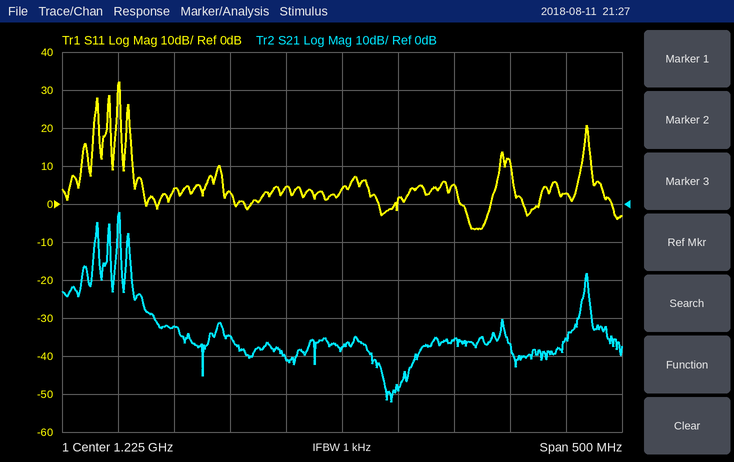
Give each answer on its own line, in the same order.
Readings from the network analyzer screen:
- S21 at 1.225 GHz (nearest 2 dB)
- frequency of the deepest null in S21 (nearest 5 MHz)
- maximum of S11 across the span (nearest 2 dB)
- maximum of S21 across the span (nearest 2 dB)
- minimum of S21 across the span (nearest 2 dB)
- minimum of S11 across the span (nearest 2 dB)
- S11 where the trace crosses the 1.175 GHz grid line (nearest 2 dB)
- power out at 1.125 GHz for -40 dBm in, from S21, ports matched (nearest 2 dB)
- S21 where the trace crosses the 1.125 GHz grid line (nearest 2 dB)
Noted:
-38 dB
1.270 GHz
32 dB
-2 dB
-52 dB
-6 dB
4 dB
-74 dBm
-34 dB
